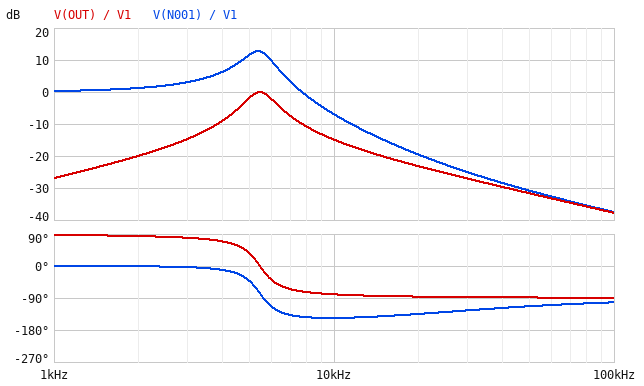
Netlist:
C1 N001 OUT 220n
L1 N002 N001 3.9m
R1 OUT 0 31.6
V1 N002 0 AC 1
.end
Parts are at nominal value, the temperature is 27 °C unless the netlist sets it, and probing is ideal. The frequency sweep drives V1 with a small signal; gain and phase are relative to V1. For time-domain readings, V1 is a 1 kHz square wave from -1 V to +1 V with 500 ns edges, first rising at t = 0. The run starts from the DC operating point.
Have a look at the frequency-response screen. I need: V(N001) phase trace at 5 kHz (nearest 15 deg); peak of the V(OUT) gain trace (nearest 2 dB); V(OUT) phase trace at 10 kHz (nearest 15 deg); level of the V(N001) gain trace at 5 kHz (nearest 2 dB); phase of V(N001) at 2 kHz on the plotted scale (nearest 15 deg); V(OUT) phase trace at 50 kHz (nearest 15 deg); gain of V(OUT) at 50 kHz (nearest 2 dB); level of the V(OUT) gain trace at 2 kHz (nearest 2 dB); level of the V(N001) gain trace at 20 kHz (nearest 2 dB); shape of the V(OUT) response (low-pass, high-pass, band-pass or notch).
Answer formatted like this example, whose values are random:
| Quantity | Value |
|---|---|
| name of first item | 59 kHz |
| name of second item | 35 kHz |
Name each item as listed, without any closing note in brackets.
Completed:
| Quantity | Value |
|---|---|
| V(N001) phase trace at 5 kHz | -45 deg |
| peak of the V(OUT) gain trace | 0 dB |
| V(OUT) phase trace at 10 kHz | -75 deg |
| level of the V(N001) gain trace at 5 kHz | 12 dB |
| phase of V(N001) at 2 kHz on the plotted scale | 0 deg |
| V(OUT) phase trace at 50 kHz | -90 deg |
| gain of V(OUT) at 50 kHz | -32 dB |
| level of the V(OUT) gain trace at 2 kHz | -20 dB |
| level of the V(N001) gain trace at 20 kHz | -20 dB |
| shape of the V(OUT) response | band-pass |
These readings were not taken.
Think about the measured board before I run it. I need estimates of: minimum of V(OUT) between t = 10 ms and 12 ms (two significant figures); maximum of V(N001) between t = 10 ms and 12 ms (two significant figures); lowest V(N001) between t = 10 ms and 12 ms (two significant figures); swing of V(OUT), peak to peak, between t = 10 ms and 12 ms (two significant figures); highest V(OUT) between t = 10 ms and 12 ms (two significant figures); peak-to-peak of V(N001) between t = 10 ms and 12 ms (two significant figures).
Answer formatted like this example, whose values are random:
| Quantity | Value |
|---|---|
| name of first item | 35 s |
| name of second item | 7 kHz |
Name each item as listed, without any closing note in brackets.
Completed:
| Quantity | Value |
|---|---|
| minimum of V(OUT) between t = 10 ms and 12 ms | -420 mV |
| maximum of V(N001) between t = 10 ms and 12 ms | 2.5 V |
| lowest V(N001) between t = 10 ms and 12 ms | -2.5 V |
| swing of V(OUT), peak to peak, between t = 10 ms and 12 ms | 840 mV |
| highest V(OUT) between t = 10 ms and 12 ms | 420 mV |
| peak-to-peak of V(N001) between t = 10 ms and 12 ms | 5.0 V |
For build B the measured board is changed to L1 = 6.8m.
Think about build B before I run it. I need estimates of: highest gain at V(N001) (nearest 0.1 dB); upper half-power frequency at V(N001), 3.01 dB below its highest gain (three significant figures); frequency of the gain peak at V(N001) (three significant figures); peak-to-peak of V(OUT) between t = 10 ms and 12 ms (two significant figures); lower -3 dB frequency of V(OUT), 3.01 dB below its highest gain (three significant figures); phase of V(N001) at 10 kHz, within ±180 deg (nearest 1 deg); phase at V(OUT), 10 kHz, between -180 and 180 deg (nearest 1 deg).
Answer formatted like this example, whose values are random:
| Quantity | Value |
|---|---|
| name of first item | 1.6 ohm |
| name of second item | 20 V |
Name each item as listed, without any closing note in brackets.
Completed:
| Quantity | Value |
|---|---|
| highest gain at V(N001) | 15.1 dB |
| upper half-power frequency at V(N001), 3.01 dB below its highest gain | 4.44 kHz |
| frequency of the gain peak at V(N001) | 4.08 kHz |
| peak-to-peak of V(OUT) between t = 10 ms and 12 ms | 480 mV |
| lower -3 dB frequency of V(OUT), 3.01 dB below its highest gain | 3.76 kHz |
| phase of V(N001) at 10 kHz, within ±180 deg | -151 deg |
| phase at V(OUT), 10 kHz, between -180 and 180 deg | -85 deg |
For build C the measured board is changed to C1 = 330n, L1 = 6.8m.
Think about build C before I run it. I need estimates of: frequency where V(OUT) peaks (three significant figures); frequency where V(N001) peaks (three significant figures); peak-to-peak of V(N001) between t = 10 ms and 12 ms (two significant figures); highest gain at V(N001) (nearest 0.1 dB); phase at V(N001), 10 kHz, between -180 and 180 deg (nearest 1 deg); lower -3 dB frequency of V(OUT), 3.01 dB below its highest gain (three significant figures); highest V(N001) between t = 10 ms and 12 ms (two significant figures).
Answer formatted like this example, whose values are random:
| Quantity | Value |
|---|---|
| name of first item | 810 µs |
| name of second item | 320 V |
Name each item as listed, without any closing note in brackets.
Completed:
| Quantity | Value |
|---|---|
| frequency where V(OUT) peaks | 3.36 kHz |
| frequency where V(N001) peaks | 3.32 kHz |
| peak-to-peak of V(N001) between t = 10 ms and 12 ms | 5.4 V |
| highest gain at V(N001) | 13.4 dB |
| phase at V(N001), 10 kHz, between -180 and 180 deg | -142 deg |
| lower -3 dB frequency of V(OUT), 3.01 dB below its highest gain | 3.01 kHz |
| highest V(N001) between t = 10 ms and 12 ms | 2.7 V |
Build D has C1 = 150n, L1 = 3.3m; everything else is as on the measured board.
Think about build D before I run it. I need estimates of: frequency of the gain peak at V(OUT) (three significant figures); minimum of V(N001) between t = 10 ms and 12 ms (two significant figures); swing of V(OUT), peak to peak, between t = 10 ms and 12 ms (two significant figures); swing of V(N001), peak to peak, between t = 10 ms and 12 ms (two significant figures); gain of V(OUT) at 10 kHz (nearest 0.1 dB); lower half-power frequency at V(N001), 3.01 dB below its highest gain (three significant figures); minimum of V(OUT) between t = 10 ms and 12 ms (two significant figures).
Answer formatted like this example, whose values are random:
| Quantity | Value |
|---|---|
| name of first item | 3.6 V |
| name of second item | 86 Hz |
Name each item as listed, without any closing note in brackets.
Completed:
| Quantity | Value |
|---|---|
| frequency of the gain peak at V(OUT) | 7.15 kHz |
| minimum of V(N001) between t = 10 ms and 12 ms | -2.6 V |
| swing of V(OUT), peak to peak, between t = 10 ms and 12 ms | 800 mV |
| swing of V(N001), peak to peak, between t = 10 ms and 12 ms | 5.2 V |
| gain of V(OUT) at 10 kHz | -10.5 dB |
| lower half-power frequency at V(N001), 3.01 dB below its highest gain | 6.27 kHz |
| minimum of V(OUT) between t = 10 ms and 12 ms | -400 mV |
